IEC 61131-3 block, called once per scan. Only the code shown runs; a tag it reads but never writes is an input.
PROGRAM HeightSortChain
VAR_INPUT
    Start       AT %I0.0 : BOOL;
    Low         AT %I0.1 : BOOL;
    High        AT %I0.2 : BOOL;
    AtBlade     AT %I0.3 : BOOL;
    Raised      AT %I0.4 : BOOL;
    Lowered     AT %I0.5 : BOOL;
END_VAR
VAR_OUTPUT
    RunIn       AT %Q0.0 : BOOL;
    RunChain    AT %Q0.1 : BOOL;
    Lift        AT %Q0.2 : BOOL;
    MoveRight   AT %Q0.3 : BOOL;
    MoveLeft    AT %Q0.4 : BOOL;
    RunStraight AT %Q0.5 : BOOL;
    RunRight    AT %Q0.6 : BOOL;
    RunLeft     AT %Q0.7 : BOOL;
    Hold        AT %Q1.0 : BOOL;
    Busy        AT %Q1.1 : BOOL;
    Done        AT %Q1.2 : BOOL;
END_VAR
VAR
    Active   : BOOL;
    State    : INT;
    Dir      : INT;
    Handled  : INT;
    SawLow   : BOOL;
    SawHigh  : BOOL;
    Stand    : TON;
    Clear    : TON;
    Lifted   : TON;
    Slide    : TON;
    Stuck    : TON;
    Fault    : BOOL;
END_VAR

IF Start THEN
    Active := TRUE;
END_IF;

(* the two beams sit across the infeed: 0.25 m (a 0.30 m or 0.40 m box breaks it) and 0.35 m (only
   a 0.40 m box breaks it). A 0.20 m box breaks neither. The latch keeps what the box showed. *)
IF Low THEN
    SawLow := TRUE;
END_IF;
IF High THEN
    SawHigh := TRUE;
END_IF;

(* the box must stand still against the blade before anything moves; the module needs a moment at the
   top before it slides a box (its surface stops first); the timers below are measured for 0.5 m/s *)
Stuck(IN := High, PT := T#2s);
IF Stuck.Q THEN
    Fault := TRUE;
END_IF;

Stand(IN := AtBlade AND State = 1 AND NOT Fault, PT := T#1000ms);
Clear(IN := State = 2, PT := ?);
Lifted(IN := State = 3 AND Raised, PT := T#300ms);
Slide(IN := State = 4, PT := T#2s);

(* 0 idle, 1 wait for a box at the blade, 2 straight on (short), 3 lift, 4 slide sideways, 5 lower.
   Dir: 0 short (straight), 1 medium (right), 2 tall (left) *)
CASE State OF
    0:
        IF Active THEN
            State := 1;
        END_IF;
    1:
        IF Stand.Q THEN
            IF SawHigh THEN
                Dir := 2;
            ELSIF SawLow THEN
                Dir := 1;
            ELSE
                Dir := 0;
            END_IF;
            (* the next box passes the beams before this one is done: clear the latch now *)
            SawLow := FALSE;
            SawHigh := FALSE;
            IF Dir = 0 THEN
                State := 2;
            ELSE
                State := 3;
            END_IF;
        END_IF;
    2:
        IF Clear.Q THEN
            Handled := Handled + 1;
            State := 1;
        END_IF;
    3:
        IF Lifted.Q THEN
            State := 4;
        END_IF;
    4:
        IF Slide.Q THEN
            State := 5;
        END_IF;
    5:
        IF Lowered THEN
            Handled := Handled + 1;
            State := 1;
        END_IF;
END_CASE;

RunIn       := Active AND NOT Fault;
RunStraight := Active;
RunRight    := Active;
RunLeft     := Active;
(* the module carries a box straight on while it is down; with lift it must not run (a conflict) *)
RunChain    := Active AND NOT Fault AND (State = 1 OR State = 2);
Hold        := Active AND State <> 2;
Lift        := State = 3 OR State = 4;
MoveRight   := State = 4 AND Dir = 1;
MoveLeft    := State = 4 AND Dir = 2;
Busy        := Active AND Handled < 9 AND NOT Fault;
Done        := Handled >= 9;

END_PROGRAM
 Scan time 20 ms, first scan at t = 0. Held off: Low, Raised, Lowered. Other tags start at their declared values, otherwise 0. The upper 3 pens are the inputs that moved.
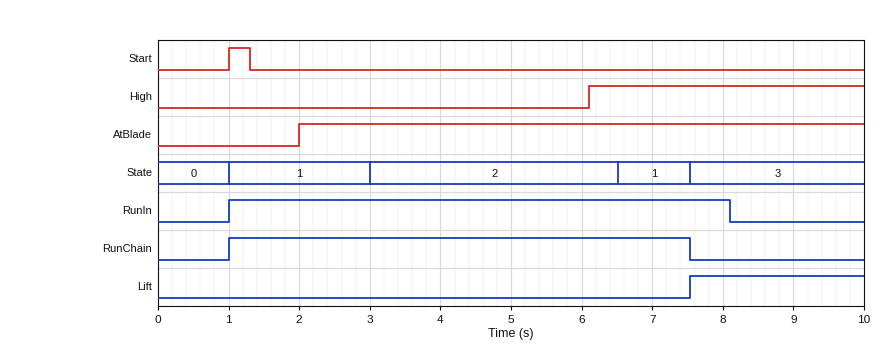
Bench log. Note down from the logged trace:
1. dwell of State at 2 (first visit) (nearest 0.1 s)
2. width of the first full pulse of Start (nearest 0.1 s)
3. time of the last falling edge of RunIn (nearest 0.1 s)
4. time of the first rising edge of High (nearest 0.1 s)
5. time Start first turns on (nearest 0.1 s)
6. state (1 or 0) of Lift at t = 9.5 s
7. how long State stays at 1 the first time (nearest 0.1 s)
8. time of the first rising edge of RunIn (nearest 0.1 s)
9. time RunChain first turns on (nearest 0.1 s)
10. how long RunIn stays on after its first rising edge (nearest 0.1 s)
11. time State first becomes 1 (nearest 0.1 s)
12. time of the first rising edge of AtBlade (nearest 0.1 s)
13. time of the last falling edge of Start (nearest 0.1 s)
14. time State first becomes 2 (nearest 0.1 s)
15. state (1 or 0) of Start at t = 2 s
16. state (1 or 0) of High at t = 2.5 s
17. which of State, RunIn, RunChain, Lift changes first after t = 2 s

3.5 s
0.3 s
8.1 s
6.1 s
1.0 s
1
2.0 s
1.0 s
1.0 s
7.1 s
1.0 s
2.0 s
1.3 s
3.0 s
0
0
State
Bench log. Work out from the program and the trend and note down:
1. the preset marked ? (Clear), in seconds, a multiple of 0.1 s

3.5 s
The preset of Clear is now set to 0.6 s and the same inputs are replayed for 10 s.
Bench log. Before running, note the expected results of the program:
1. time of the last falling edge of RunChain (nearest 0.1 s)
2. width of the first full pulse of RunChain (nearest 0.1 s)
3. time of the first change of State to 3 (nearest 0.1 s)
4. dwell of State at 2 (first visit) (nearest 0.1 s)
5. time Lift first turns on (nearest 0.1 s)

6.3 s
5.3 s
6.3 s
0.6 s
6.3 s
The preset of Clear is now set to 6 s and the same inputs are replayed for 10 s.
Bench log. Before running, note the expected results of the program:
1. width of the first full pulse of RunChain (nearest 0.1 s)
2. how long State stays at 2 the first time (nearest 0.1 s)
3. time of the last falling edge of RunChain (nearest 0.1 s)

7.1 s
6.0 s
8.1 s
